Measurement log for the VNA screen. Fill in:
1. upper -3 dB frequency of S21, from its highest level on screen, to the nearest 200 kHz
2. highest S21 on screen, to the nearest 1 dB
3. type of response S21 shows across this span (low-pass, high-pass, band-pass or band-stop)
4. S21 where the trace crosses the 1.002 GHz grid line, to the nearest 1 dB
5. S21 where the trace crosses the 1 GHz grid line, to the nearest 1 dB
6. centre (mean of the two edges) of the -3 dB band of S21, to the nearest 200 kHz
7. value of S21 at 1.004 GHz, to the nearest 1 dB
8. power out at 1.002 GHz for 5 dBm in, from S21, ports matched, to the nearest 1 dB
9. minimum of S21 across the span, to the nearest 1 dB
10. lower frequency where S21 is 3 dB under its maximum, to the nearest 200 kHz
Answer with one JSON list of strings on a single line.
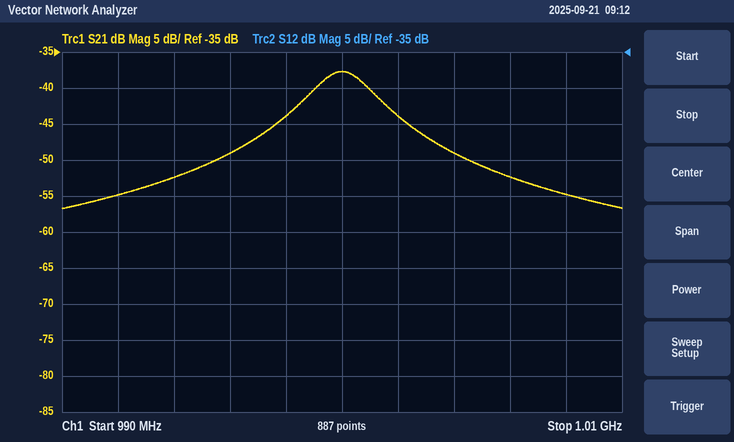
["1.0012 GHz", "-38 dB", "band-pass", "-44 dB", "-38 dB", "1.0000 GHz", "-49 dB", "-39 dBm", "-57 dB", "998.8 MHz"]
